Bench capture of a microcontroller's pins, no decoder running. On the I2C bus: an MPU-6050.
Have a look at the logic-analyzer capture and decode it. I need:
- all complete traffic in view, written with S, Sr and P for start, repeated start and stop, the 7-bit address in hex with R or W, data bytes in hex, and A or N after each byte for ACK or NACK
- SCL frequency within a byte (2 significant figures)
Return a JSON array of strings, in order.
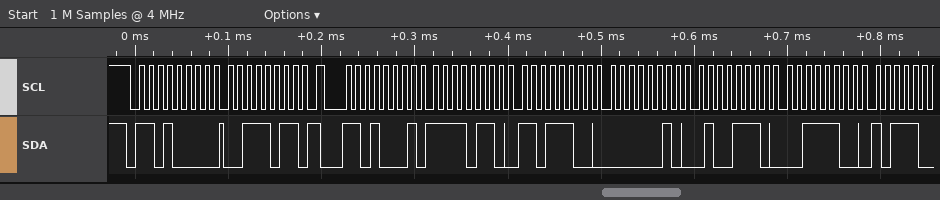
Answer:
["S 68W A 3B A Sr 68R A F6 A DC A 02 A 4E A 3C A", "100 kHz"]
